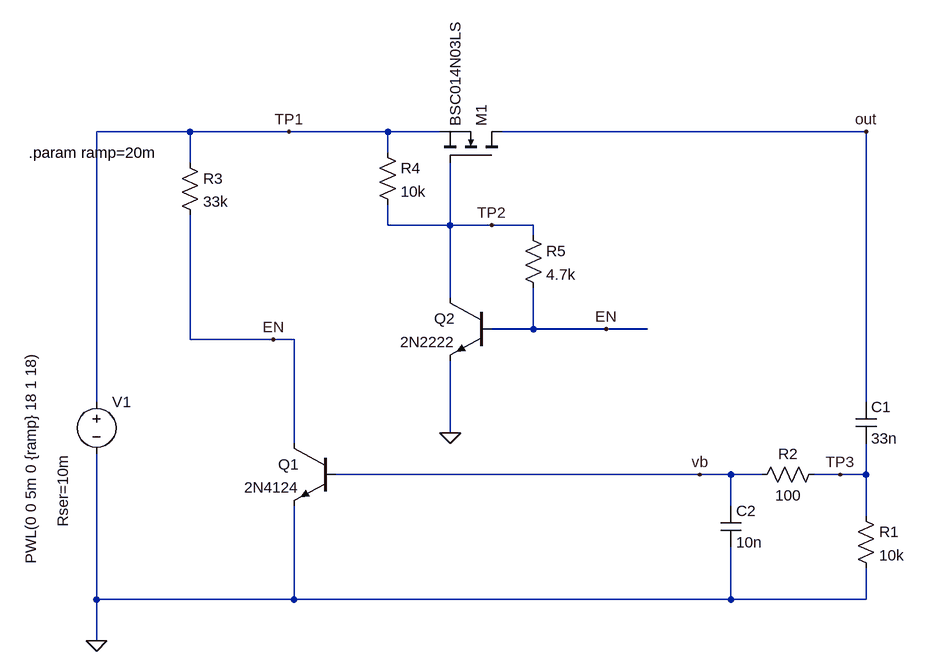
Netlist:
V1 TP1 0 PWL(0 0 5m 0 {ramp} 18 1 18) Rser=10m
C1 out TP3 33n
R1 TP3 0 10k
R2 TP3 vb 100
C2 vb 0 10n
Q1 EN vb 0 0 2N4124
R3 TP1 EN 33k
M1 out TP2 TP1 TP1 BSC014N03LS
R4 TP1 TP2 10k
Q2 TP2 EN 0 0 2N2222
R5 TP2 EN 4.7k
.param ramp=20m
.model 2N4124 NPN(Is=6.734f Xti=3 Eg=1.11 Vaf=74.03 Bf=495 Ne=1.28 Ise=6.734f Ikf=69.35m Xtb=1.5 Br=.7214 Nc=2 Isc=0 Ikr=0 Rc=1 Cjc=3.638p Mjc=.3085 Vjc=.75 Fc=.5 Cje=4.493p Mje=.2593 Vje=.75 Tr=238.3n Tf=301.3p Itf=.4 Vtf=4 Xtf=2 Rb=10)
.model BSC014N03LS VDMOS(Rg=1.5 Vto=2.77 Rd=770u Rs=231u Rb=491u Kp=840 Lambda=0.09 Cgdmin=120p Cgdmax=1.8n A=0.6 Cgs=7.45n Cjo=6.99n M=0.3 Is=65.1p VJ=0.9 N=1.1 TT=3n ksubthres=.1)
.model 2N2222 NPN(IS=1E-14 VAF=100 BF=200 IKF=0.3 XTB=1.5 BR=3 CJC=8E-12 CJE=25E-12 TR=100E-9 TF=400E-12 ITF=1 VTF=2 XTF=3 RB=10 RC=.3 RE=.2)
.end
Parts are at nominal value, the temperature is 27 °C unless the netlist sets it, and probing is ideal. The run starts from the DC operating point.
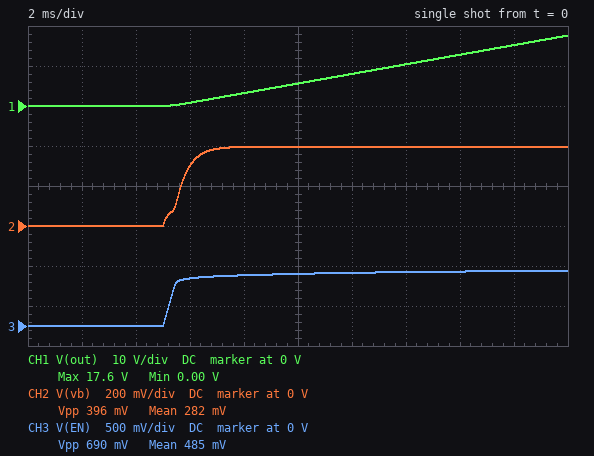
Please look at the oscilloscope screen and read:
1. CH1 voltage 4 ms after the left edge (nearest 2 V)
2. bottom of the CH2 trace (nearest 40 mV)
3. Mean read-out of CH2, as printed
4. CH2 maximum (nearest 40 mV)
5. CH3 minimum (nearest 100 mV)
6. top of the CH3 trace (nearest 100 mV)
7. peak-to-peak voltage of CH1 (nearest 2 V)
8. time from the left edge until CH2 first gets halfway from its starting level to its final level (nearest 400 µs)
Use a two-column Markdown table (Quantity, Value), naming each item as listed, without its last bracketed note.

| Quantity | Value |
|---|---|
| CH1 voltage 4 ms after the left edge | 0 V |
| bottom of the CH2 trace | 0 V |
| Mean read-out of CH2, as printed | 282 mV |
| CH2 maximum | 400 mV |
| CH3 minimum | 0 V |
| top of the CH3 trace | 700 mV |
| peak-to-peak voltage of CH1 | 18 V |
| time from the left edge until CH2 first gets halfway from its starting level to its final level | 5.6 ms |
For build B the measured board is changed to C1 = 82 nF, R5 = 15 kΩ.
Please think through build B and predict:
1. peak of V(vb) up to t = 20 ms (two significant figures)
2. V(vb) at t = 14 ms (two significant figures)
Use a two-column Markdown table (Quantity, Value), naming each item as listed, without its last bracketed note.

| Quantity | Value |
|---|---|
| peak of V(vb) up to t = 20 ms | 670 mV |
| V(vb) at t = 14 ms | 660 mV |
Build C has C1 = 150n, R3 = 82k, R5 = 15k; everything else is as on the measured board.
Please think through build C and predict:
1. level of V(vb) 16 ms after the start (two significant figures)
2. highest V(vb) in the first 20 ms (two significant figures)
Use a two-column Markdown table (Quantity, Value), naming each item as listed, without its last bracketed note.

| Quantity | Value |
|---|---|
| level of V(vb) 16 ms after the start | 660 mV |
| highest V(vb) in the first 20 ms | 670 mV |
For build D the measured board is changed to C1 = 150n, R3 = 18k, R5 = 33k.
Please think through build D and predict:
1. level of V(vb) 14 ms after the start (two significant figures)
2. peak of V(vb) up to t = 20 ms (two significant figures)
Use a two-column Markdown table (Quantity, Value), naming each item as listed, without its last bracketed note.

| Quantity | Value |
|---|---|
| level of V(vb) 14 ms after the start | 670 mV |
| peak of V(vb) up to t = 20 ms | 680 mV |
